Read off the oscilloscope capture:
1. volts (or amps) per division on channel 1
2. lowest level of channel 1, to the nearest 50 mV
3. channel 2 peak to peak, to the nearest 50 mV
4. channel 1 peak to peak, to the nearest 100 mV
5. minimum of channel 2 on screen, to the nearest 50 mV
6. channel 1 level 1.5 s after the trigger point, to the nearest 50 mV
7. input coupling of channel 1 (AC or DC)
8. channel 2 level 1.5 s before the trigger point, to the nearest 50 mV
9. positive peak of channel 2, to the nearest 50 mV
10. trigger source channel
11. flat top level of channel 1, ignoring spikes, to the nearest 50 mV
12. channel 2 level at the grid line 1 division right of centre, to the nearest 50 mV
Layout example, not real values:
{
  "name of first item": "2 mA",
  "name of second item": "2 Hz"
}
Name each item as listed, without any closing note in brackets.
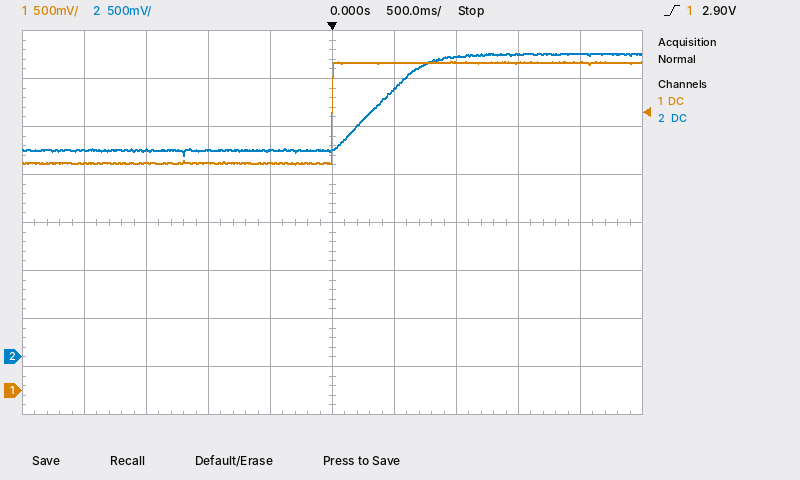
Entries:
{
  "volts (or amps) per division on channel 1": "500 mV",
  "lowest level of channel 1, to the nearest 50 mV": "2.35 V",
  "channel 2 peak to peak, to the nearest 50 mV": "1.05 V",
  "channel 1 peak to peak, to the nearest 100 mV": "1.10 V",
  "minimum of channel 2 on screen, to the nearest 50 mV": "2.10 V",
  "channel 1 level 1.5 s after the trigger point, to the nearest 50 mV": "3.40 V",
  "input coupling of channel 1": "DC",
  "channel 2 level 1.5 s before the trigger point, to the nearest 50 mV": "2.15 V",
  "positive peak of channel 2, to the nearest 50 mV": "3.15 V",
  "trigger source channel": "channel 1",
  "flat top level of channel 1, ignoring spikes, to the nearest 50 mV": "3.40 V",
  "channel 2 level at the grid line 1 division right of centre, to the nearest 50 mV": "2.80 V"
}
